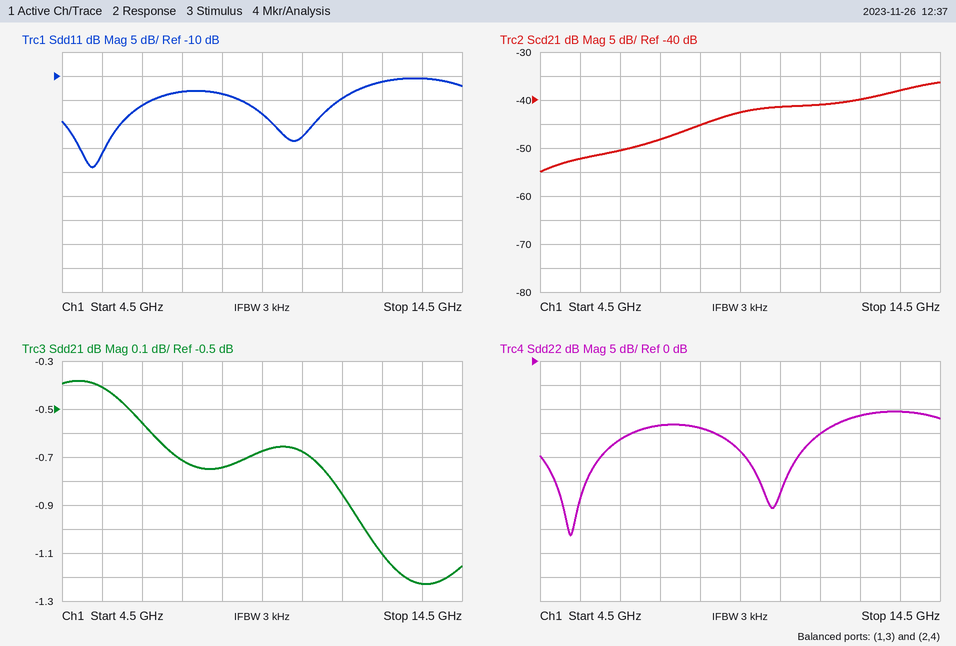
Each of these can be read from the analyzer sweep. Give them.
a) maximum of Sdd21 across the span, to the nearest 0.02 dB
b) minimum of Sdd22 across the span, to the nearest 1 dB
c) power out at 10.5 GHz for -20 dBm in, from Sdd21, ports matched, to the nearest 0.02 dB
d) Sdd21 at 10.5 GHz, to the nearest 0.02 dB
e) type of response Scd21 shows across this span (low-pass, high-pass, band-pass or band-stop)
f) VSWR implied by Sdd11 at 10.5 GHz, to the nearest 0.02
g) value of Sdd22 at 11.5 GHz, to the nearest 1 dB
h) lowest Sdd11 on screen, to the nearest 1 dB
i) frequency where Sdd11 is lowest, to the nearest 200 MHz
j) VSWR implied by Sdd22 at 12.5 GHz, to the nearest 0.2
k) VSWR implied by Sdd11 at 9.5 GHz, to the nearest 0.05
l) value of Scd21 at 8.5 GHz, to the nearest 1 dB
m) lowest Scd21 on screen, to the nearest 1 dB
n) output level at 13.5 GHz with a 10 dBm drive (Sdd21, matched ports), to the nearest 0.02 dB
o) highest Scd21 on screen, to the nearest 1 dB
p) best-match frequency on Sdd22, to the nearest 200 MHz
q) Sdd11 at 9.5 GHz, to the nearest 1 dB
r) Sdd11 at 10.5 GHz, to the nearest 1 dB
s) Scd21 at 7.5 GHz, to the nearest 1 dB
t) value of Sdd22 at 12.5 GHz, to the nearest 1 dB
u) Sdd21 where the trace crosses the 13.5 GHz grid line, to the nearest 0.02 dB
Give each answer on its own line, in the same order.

-0.38 dB
-36 dB
-20.68 dBm
-0.68 dB
high-pass
1.16
-15 dB
-29 dB
5.2 GHz
1.8
1.30
-45 dB
-55 dB
8.78 dBm
-36 dB
5.2 GHz
-18 dB
-23 dB
-48 dB
-11 dB
-1.22 dB
